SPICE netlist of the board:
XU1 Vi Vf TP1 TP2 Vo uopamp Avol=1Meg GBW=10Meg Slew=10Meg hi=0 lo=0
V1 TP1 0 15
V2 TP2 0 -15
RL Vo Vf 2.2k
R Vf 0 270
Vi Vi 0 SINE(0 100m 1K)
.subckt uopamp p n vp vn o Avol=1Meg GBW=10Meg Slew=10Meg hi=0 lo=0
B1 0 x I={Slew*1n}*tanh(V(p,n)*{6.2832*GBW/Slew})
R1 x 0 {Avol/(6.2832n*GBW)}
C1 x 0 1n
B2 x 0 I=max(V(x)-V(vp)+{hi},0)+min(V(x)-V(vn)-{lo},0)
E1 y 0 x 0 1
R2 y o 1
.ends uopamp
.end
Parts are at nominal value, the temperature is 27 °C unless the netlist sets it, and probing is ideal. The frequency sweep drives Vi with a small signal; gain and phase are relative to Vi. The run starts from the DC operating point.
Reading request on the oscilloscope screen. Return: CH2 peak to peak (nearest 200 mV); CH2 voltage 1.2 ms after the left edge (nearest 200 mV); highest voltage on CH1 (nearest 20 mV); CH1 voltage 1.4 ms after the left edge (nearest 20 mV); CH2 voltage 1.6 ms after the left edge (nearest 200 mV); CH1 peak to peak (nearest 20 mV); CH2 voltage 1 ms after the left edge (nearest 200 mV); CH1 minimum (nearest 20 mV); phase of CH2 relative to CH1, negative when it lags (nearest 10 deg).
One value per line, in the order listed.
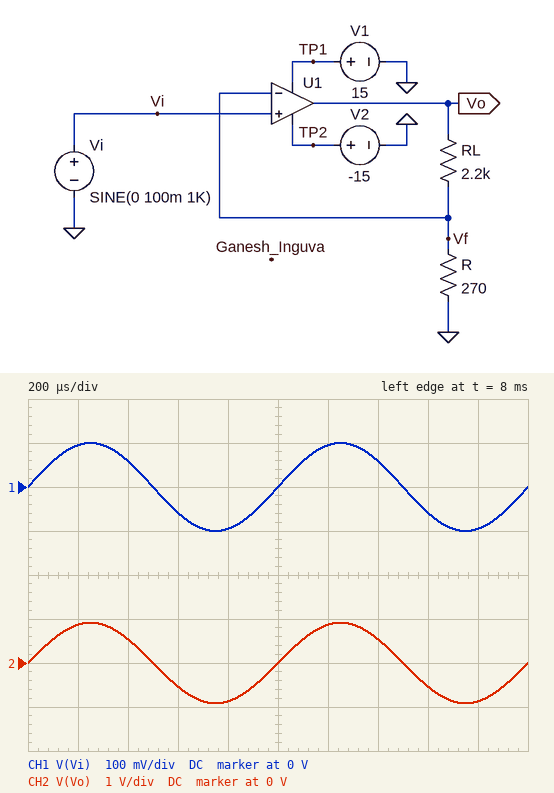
1.8 V
800 mV
100 mV
60 mV
-600 mV
200 mV
0 V
-100 mV
0 deg
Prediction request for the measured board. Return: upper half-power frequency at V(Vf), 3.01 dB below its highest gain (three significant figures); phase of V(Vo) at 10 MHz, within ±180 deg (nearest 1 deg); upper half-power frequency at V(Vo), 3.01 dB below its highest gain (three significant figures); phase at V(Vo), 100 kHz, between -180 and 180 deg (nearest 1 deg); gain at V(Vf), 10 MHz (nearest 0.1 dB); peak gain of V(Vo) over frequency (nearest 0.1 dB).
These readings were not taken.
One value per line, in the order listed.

1.09 MHz
-84 deg
1.09 MHz
-5 deg
-19.3 dB
19.2 dB
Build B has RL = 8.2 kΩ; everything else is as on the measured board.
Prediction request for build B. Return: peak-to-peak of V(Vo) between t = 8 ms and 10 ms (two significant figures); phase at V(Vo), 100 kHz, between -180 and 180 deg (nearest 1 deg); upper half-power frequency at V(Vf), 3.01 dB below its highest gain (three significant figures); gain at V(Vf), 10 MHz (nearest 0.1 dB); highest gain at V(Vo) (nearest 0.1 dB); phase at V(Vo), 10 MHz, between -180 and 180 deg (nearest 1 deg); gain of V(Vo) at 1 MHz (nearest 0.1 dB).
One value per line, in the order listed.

6.3 V
-17 deg
319 kHz
-29.9 dB
29.9 dB
-88 deg
19.6 dB
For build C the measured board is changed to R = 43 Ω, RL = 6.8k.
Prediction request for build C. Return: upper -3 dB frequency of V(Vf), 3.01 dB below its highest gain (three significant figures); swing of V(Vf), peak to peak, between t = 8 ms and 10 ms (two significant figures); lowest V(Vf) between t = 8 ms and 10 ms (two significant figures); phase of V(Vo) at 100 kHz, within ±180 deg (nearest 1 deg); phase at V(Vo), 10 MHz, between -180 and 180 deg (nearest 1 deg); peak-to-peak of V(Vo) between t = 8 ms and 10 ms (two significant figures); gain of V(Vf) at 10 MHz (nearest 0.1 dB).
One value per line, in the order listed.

62.8 kHz
190 mV
-94 mV
-58 deg
-90 deg
30 V
-44.0 dB
